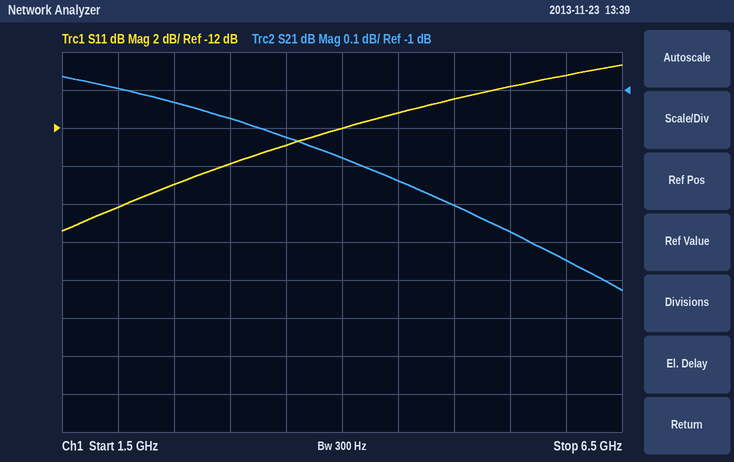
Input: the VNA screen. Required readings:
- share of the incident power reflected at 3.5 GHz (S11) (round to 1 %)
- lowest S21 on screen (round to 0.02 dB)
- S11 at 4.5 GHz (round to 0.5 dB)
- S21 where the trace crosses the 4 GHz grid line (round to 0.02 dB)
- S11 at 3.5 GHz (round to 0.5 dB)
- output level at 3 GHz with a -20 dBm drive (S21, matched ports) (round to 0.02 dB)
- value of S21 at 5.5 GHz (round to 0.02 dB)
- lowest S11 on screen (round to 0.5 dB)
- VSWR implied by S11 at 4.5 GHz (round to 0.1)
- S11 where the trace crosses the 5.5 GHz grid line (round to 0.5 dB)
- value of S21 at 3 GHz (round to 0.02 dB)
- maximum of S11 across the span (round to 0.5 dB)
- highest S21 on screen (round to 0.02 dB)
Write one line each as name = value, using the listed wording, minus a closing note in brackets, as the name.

share of the incident power reflected at 3.5 GHz (S11) = 5 %
lowest S21 on screen = -1.52 dB
S11 at 4.5 GHz = -11.0 dB
S21 where the trace crosses the 4 GHz grid line = -1.18 dB
S11 at 3.5 GHz = -13.0 dB
output level at 3 GHz with a -20 dBm drive (S21, matched ports) = -21.08 dBm
value of S21 at 5.5 GHz = -1.38 dB
lowest S11 on screen = -17.5 dB
VSWR implied by S11 at 4.5 GHz = 1.8
S11 where the trace crosses the 5.5 GHz grid line = -10.0 dB
value of S21 at 3 GHz = -1.08 dB
maximum of S11 across the span = -8.5 dB
highest S21 on screen = -0.96 dB
